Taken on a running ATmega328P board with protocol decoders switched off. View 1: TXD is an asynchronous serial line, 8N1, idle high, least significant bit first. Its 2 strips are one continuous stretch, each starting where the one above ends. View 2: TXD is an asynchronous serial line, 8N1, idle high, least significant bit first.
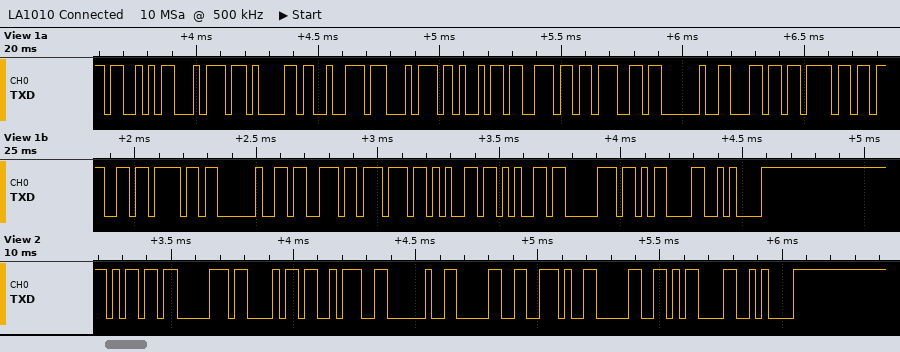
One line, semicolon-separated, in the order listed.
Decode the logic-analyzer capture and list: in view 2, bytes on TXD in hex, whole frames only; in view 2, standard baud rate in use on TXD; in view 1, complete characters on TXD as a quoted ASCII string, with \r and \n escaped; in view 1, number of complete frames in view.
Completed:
0x6D 0x70 0x68 0x3A 0x20 0x30 0x2E 0x30 0x0D 0x0A; 38400 baud; "Starting logo sweep\r\n"; 21
